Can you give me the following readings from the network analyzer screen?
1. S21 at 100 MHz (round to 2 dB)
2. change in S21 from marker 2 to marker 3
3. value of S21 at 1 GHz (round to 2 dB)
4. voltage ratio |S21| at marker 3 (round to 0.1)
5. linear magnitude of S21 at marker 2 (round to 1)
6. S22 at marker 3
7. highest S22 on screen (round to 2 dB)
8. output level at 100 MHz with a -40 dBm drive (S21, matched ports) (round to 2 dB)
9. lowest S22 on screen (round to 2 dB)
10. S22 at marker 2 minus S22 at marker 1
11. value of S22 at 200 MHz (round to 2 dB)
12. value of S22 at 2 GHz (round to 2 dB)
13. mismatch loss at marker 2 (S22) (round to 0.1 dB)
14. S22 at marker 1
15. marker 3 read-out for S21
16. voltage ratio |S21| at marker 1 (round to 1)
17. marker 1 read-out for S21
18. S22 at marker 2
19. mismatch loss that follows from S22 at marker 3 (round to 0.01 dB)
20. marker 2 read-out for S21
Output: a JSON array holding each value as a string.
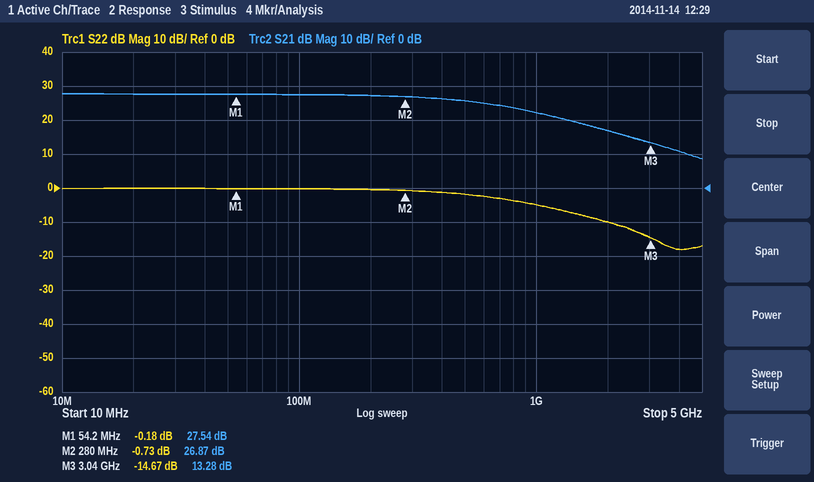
["28 dB", "-13.59 dB", "22 dB", "4.6", "22", "-14.67 dB", "0 dB", "-12 dBm", "-18 dB", "-0.55 dB", "0 dB", "-10 dB", "8.1 dB", "-0.18 dB", "13.28 dB", "24", "27.54 dB", "-0.73 dB", "0.15 dB", "26.87 dB"]
